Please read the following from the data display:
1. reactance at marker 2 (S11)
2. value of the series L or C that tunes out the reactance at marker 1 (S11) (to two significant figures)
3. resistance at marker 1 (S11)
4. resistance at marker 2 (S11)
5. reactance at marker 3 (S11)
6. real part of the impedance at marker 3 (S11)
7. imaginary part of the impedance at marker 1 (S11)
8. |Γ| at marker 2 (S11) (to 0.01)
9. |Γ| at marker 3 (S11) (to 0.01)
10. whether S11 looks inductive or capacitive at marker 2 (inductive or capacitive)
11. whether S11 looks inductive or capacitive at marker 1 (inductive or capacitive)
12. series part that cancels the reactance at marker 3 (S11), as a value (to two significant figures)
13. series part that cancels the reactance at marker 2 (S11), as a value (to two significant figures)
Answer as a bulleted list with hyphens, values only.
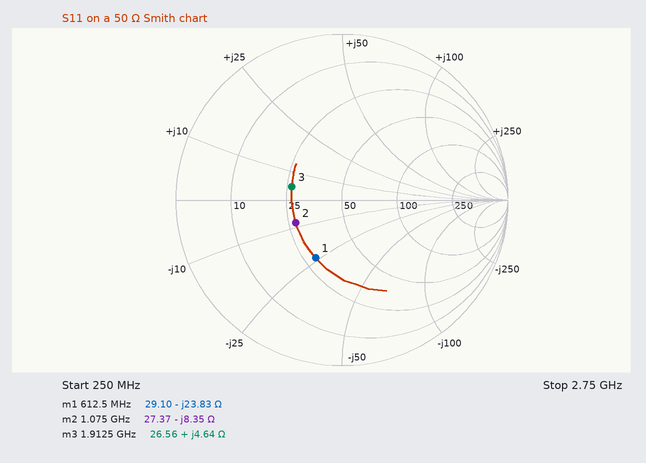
- -8.35 Ω
- 6.2 nH
- 29.10 Ω
- 27.37 Ω
- +4.64 Ω
- 26.56 Ω
- -23.83 Ω
- 0.31
- 0.31
- capacitive
- capacitive
- 18 pF
- 1.2 nH
